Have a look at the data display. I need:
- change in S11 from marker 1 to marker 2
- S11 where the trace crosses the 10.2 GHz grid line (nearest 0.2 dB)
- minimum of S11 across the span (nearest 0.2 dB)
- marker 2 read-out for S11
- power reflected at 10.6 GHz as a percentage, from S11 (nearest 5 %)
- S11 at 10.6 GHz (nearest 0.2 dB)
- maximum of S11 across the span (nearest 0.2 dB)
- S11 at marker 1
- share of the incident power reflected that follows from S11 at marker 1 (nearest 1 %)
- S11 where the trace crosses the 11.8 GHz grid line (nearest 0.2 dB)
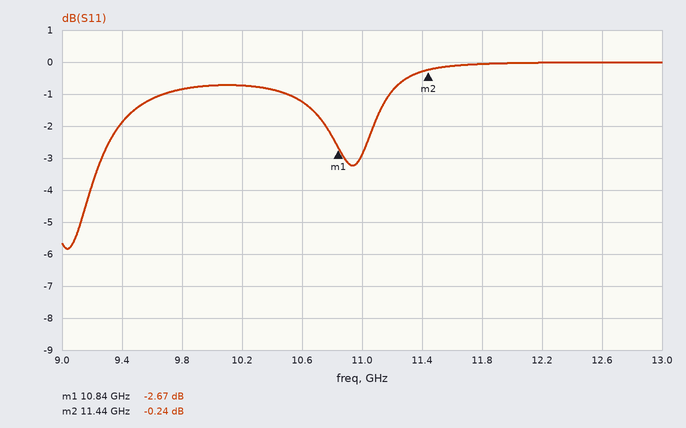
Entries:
2.43 dB
-0.8 dB
-5.8 dB
-0.24 dB
75 %
-1.2 dB
0.0 dB
-2.67 dB
54 %
0.0 dB
